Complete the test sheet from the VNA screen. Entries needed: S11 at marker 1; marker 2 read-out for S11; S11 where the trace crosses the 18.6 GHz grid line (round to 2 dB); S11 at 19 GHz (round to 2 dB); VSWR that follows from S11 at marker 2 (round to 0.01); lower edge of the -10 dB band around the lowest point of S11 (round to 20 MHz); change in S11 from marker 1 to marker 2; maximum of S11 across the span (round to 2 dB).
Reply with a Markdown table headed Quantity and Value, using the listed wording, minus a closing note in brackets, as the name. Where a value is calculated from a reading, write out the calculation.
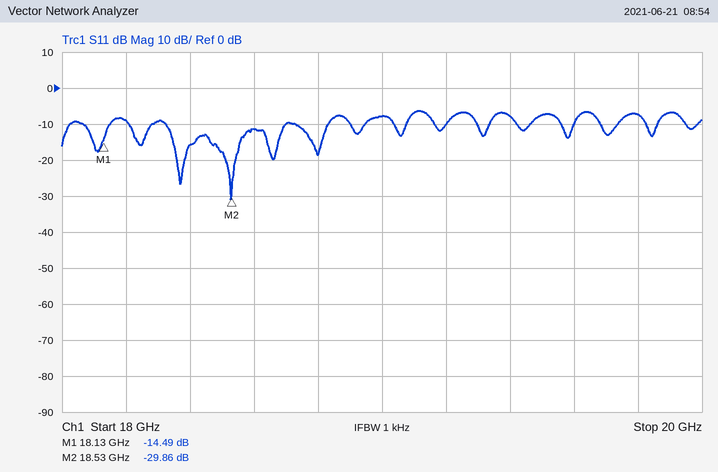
| Quantity | Value |
|---|---|
| S11 at marker 1 | -14.49 dB |
| marker 2 read-out for S11 | -29.86 dB |
| S11 where the trace crosses the 18.6 GHz grid line | -12 dB |
| S11 at 19 GHz | -8 dB |
| VSWR that follows from S11 at marker 2 | (1 + 0.0321)/(1 − 0.0321) ≈ 1.07 |
| lower edge of the -10 dB band around the lowest point of S11 | 18.32 GHz |
| change in S11 from marker 1 to marker 2 | -29.86 − (-14.49) = -15.37 dB |
| maximum of S11 across the span | -6 dB |
